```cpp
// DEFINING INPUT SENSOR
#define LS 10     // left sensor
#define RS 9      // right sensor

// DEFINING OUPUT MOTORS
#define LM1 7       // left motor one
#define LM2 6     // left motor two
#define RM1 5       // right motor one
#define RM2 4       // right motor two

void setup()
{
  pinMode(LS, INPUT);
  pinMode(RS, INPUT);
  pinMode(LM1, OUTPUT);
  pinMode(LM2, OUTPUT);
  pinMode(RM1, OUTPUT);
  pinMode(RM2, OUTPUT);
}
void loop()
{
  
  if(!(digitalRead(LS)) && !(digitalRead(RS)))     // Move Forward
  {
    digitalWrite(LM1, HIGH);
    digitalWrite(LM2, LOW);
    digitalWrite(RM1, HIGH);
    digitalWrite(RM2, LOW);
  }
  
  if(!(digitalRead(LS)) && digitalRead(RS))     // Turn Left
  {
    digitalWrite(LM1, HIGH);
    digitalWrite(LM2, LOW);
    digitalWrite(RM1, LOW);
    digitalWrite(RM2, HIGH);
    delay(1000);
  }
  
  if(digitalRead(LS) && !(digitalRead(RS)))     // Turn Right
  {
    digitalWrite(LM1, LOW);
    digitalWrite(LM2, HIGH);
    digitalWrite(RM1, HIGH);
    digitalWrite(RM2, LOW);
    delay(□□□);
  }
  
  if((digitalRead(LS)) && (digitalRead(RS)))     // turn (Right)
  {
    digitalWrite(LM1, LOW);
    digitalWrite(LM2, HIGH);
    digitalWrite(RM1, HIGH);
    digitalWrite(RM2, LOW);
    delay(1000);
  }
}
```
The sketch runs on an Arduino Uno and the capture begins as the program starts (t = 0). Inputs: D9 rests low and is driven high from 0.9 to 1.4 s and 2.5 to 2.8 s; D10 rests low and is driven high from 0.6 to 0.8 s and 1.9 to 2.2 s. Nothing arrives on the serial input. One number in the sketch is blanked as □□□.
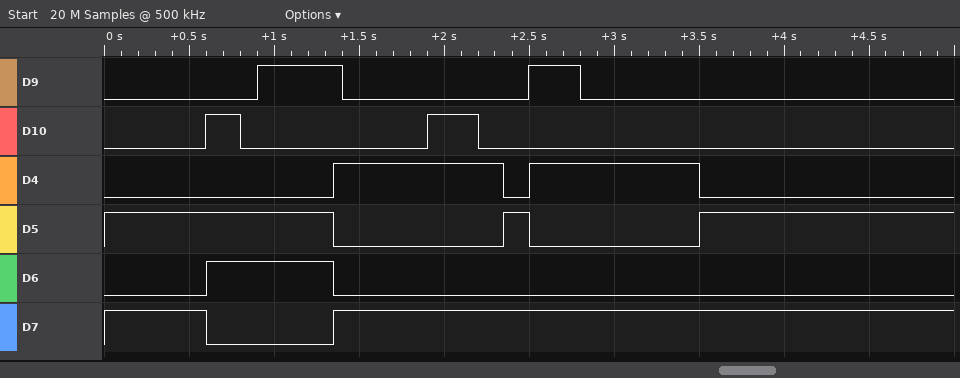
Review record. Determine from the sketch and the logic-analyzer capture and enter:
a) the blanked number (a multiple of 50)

750
